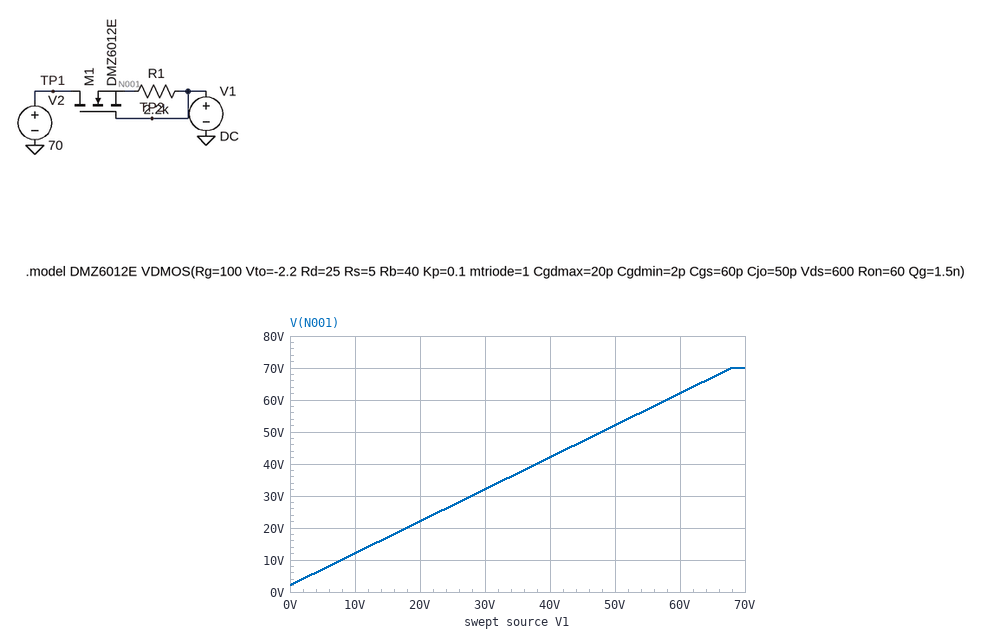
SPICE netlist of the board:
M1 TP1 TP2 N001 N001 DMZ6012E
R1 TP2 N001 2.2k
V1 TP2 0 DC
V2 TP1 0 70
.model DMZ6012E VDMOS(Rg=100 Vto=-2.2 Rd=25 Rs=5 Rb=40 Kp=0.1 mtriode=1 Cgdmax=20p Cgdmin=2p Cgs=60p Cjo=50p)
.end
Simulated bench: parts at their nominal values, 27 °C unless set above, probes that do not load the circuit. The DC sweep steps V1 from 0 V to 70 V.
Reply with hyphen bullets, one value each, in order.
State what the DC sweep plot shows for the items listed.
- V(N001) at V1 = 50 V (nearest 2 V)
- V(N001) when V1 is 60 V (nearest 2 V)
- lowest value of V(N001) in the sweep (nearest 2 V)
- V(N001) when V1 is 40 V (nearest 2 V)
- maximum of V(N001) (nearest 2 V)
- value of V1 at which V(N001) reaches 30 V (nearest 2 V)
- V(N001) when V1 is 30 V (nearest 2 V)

- 52 V
- 62 V
- 2 V
- 42 V
- 70 V
- 28 V
- 32 V
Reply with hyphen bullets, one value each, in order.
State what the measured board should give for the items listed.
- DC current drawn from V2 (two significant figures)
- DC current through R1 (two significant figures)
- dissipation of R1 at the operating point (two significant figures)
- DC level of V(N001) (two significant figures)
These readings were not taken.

- 950 µA
- 950 µA
- 2.0 mW
- 2.1 V
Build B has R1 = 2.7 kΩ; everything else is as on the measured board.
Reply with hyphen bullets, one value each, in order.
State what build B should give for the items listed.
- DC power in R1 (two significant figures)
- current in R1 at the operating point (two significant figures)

- 1.6 mW
- 780 µA
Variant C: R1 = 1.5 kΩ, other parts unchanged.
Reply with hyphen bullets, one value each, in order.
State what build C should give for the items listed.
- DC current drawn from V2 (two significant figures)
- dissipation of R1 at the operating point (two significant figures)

- 1.4 mA
- 2.8 mW
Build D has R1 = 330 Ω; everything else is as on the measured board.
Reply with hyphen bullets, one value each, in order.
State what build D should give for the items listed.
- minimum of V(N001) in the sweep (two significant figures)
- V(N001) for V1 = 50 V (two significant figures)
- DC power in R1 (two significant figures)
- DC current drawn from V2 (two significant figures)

- 1.8 V
- 52 V
- 10 mW
- 5.6 mA
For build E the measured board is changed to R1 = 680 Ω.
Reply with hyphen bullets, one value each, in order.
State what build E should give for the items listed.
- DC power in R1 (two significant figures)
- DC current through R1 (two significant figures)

- 5.6 mW
- 2.9 mA
